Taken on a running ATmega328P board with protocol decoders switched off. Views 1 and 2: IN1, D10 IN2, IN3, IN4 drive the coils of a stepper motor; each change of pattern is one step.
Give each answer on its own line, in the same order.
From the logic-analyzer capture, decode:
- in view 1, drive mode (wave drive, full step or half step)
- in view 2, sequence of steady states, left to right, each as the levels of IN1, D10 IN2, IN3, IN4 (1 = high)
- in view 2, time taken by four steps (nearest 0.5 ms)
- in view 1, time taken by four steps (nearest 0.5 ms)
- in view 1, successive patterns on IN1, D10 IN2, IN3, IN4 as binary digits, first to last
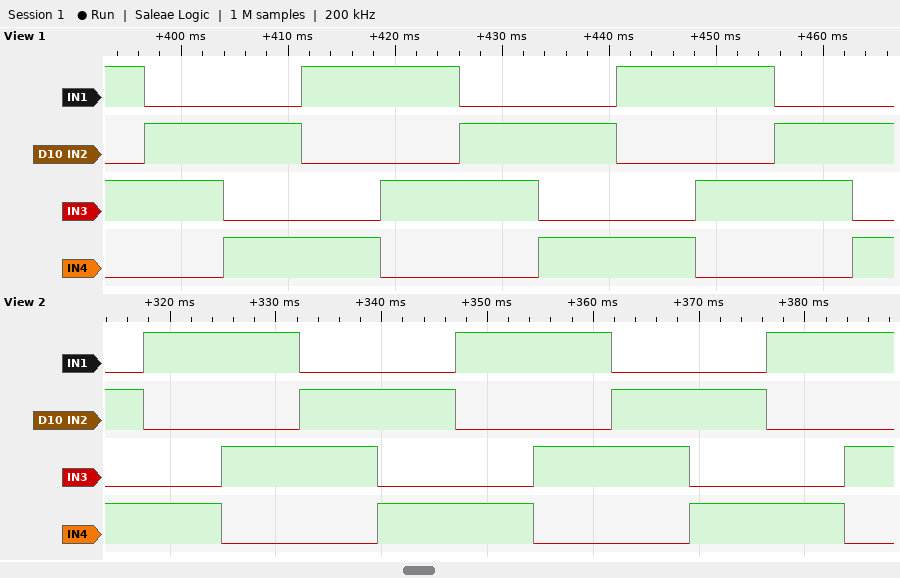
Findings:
full step
0101 1001 1010 0110 0101 1001 1010 0110 0101 1001 1010
29.5 ms
29.5 ms
1010 0110 0101 1001 1010 0110 0101 1001 1010 0110 0101
